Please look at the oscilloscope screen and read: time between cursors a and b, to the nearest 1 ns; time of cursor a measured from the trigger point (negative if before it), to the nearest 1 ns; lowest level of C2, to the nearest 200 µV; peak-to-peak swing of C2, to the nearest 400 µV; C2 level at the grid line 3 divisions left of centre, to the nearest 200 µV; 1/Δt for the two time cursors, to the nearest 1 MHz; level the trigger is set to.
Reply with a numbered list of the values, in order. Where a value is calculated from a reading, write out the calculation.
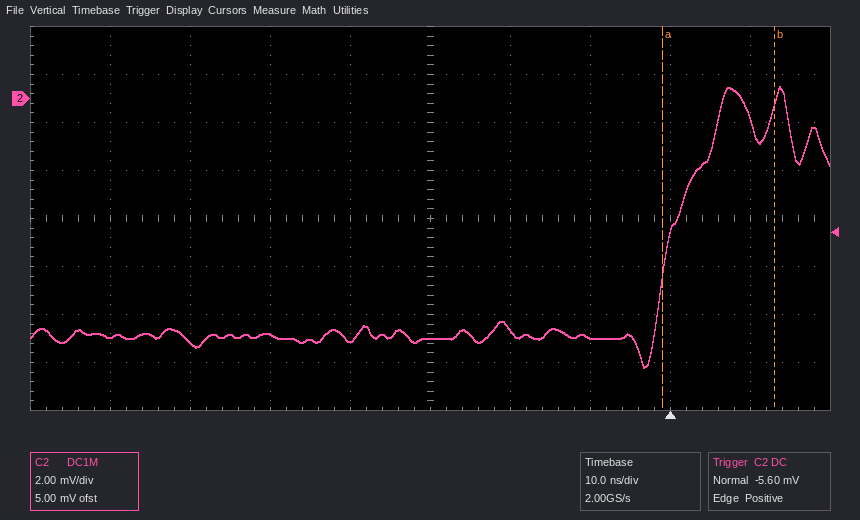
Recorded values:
1. 14 ns
2. -1 ns
3. -11.2 mV
4. 11.6 mV
5. -10.2 mV
6. 1 / 14 ns ≈ 71 MHz
7. -5.60 mV
